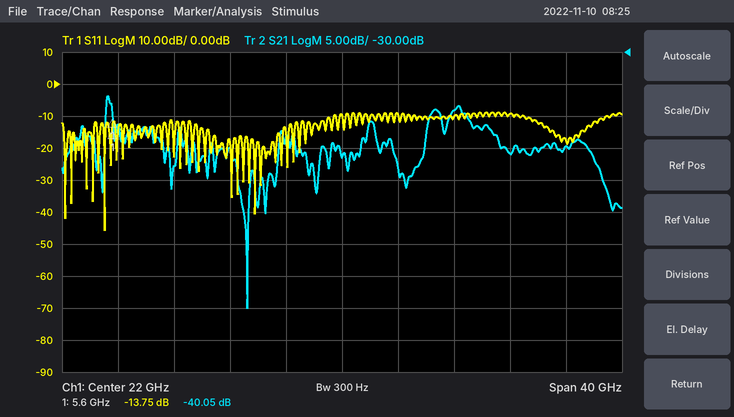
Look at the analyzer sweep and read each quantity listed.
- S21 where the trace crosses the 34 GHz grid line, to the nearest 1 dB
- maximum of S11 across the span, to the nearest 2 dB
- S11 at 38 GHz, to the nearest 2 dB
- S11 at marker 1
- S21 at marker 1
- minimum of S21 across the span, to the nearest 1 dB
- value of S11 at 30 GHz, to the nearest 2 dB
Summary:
-46 dB
-8 dB
-18 dB
-13.75 dB
-40.05 dB
-70 dB
-10 dB
